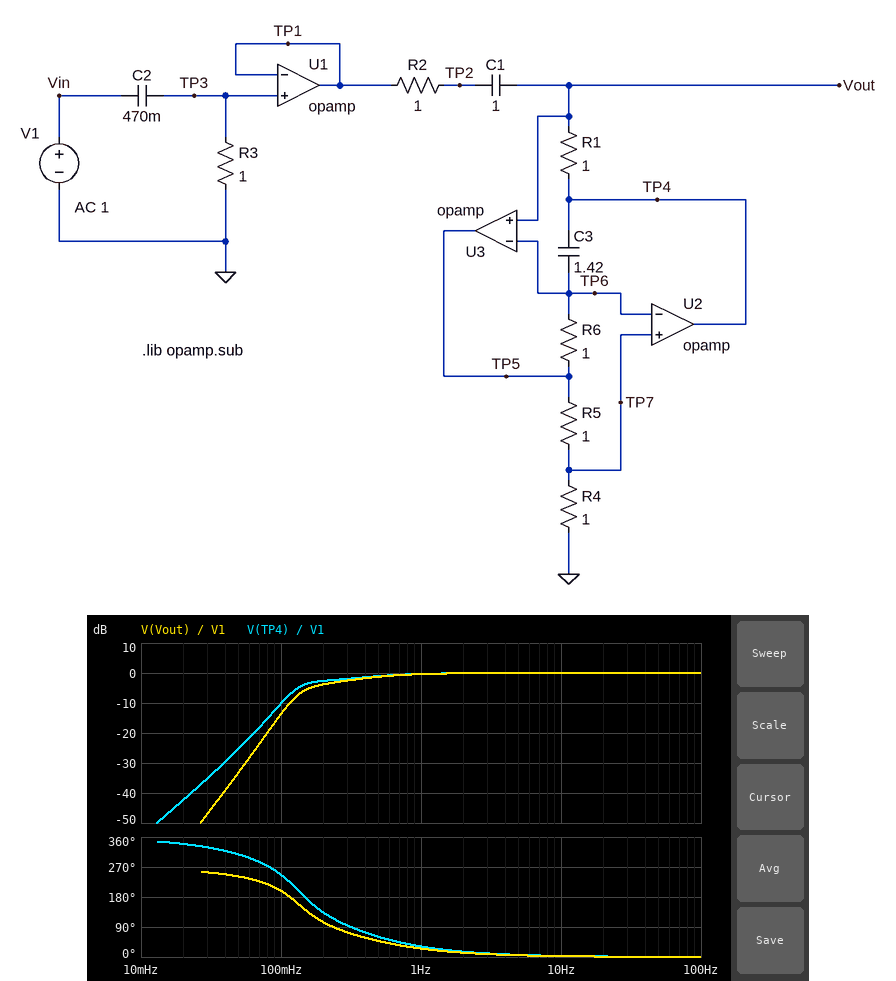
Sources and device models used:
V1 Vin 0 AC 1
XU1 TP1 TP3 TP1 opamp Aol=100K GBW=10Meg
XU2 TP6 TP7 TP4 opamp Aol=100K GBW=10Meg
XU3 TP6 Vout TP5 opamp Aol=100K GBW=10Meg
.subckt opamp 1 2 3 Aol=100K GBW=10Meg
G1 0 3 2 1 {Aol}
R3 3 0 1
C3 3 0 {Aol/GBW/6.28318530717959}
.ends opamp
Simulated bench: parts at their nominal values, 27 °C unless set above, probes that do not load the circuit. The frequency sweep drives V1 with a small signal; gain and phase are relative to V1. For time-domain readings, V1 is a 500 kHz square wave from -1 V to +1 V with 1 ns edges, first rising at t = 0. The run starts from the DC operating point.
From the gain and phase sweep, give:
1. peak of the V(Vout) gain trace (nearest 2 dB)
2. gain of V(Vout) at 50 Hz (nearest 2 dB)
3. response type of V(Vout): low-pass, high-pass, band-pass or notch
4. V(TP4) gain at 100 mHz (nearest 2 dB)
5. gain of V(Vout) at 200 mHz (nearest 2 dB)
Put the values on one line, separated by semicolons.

0 dB; 0 dB; high-pass; -10 dB; -4 dB
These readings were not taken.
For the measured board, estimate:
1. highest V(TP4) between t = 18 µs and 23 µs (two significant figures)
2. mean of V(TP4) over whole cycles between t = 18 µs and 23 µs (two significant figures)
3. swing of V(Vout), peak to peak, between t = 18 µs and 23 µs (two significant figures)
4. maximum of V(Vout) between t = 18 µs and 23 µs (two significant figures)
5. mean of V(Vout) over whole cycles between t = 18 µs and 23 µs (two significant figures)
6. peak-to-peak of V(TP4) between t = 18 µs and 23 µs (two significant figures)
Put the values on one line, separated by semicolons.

2.0 V; 1.0 V; 2.0 V; 2.0 V; 1.0 V; 2.0 V
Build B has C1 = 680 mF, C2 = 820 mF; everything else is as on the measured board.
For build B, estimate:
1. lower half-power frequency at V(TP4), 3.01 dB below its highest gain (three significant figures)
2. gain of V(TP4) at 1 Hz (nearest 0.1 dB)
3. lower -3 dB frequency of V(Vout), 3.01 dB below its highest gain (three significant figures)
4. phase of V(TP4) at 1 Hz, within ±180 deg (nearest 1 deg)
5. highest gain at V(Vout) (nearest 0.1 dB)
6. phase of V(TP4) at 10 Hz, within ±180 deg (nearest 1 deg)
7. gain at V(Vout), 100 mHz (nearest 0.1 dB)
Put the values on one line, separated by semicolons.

142 mHz; 0.1 dB; 148 mHz; 24 deg; 0.8 dB; 2 deg; -12.7 dB
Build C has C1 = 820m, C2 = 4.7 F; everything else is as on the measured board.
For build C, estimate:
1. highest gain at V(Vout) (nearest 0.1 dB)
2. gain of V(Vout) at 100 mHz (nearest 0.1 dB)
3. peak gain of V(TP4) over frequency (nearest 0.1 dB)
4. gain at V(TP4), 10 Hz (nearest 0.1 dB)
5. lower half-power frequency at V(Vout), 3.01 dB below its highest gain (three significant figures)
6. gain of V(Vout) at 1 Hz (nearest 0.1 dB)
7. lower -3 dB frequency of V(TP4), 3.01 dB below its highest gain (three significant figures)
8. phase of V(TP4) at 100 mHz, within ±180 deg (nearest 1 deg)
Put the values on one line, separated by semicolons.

2.9 dB; -4.7 dB; 4.5 dB; 0 dB; 125 mHz; 0.1 dB; 117 mHz; -157 deg
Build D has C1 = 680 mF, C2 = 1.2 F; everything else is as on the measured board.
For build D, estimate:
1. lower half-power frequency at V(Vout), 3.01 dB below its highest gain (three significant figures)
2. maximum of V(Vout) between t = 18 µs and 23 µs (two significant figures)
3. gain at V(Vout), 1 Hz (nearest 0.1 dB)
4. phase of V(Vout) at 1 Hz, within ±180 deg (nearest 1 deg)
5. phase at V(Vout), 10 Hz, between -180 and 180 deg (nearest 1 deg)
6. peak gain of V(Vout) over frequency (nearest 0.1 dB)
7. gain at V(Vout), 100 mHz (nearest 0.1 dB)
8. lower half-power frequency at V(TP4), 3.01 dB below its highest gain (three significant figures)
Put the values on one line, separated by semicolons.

144 mHz; 2.0 V; 0.1 dB; 14 deg; 1 deg; 2.1 dB; -10.3 dB; 138 mHz
